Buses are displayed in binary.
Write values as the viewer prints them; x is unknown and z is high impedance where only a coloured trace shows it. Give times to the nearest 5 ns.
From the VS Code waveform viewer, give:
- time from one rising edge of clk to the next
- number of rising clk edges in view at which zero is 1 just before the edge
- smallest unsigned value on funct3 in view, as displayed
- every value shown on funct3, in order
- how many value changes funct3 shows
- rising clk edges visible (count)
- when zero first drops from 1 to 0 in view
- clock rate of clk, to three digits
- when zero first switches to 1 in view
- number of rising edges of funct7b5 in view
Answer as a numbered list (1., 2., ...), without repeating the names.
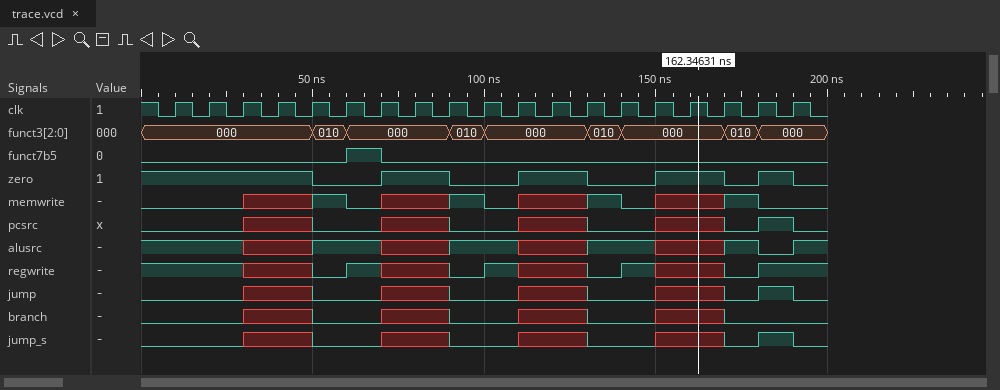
1. 10 ns
2. 12
3. 000
4. 000, 010, 000, 010, 000, 010, 000, 010, 000
5. 8
6. 19
7. 50 ns
8. 100 MHz
9. 70 ns
10. 1
